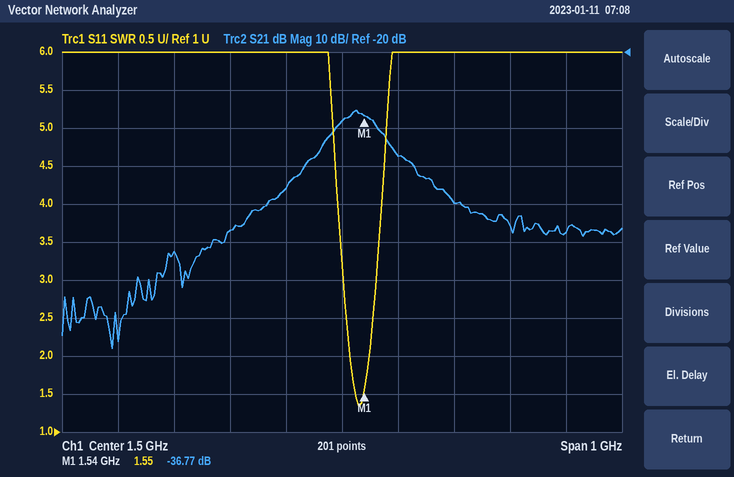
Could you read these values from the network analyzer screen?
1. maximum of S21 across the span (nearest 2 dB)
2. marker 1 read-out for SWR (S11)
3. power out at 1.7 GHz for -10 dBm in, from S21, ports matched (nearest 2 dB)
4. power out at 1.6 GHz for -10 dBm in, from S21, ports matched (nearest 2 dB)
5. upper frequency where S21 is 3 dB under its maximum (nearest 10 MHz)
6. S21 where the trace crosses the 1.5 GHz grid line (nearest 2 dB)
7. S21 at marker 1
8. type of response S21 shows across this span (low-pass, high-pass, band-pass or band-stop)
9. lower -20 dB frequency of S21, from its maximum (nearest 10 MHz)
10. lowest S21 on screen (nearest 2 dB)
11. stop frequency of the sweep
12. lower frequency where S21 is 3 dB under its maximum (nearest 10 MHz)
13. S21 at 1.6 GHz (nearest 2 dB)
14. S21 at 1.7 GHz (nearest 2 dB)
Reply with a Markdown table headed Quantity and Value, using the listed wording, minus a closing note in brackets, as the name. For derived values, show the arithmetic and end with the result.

| Quantity | Value |
|---|---|
| maximum of S21 across the span | -36 dB |
| marker 1 read-out for SWR | 1.55 |
| power out at 1.7 GHz for -10 dBm in, from S21, ports matched | -10 dBm + (-60 dB) = -70 dBm |
| power out at 1.6 GHz for -10 dBm in, from S21, ports matched | -10 dBm + (-48 dB) = -58 dBm |
| upper frequency where S21 is 3 dB under its maximum | 1.56 GHz |
| S21 where the trace crosses the 1.5 GHz grid line | -38 dB |
| S21 at marker 1 | -36.77 dB |
| type of response S21 shows across this span | band-pass |
| lower -20 dB frequency of S21, from its maximum | 1.40 GHz |
| lowest S21 on screen | -98 dB |
| stop frequency of the sweep | 2 GHz |
| lower frequency where S21 is 3 dB under its maximum | 1.50 GHz |
| S21 at 1.6 GHz | -48 dB |
| S21 at 1.7 GHz | -60 dB |
